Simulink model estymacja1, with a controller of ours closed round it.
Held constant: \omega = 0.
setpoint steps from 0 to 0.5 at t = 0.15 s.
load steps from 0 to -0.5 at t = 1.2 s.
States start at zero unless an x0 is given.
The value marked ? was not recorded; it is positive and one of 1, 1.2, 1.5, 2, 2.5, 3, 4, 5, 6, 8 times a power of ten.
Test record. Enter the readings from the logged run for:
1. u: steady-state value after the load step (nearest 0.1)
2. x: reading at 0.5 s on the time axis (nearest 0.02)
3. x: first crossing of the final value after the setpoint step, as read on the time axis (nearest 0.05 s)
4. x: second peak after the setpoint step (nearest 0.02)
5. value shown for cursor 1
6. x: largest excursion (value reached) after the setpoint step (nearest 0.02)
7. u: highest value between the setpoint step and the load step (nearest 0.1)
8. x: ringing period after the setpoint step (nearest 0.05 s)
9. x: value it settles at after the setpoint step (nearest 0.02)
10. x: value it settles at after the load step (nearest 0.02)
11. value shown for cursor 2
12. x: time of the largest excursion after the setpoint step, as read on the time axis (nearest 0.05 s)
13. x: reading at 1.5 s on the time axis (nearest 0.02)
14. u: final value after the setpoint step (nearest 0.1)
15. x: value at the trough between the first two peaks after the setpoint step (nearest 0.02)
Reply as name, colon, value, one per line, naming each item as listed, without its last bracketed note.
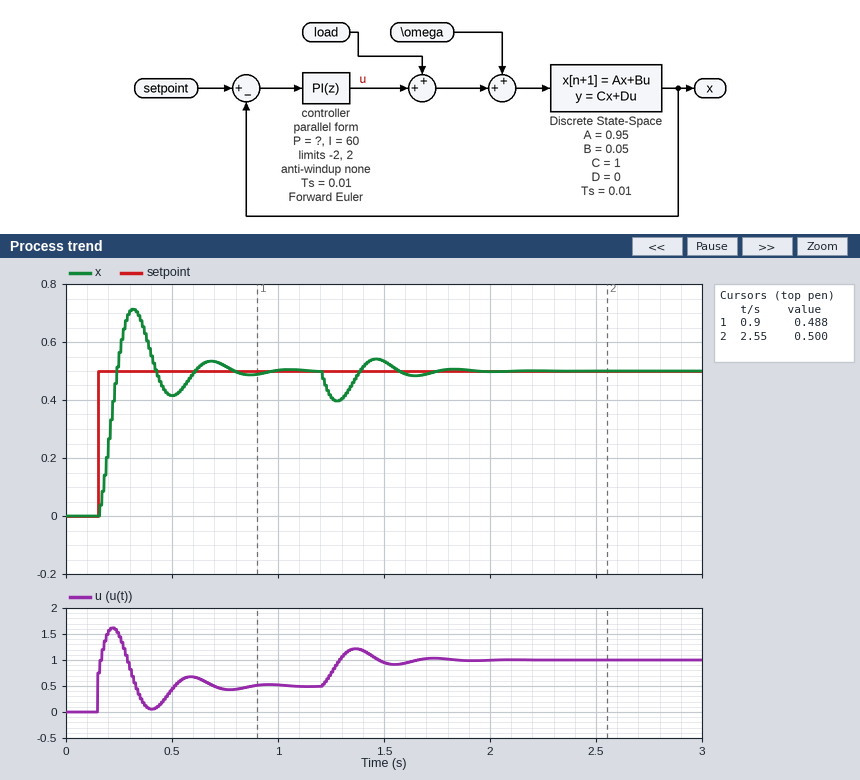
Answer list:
u: steady-state value after the load step: 1.0
x: reading at 0.5 s on the time axis: 0.42
x: first crossing of the final value after the setpoint step, as read on the time axis: 0.25 s
x: second peak after the setpoint step: 0.54
value shown for cursor 1: 0.488
x: largest excursion (value reached) after the setpoint step: 0.72
u: highest value between the setpoint step and the load step: 1.6
x: ringing period after the setpoint step: 0.35 s
x: value it settles at after the setpoint step: 0.50
x: value it settles at after the load step: 0.50
value shown for cursor 2: 0.500
x: time of the largest excursion after the setpoint step, as read on the time axis: 0.30 s
x: reading at 1.5 s on the time axis: 0.54
u: final value after the setpoint step: 0.5
x: value at the trough between the first two peaks after the setpoint step: 0.42
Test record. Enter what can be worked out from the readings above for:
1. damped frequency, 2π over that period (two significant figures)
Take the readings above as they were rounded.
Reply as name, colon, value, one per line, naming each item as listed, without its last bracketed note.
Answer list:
damped frequency, 2π over that period: 18 rad/s
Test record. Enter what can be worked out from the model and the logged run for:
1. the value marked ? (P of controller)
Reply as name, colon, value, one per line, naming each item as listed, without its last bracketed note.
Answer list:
the value marked ?: 1.5
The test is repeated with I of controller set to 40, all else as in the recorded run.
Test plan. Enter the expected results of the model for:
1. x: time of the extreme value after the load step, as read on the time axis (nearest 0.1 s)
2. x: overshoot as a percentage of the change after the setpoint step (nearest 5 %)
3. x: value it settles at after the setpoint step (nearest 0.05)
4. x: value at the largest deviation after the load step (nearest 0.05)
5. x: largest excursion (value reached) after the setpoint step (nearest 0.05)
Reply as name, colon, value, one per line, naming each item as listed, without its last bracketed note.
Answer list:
x: time of the extreme value after the load step, as read on the time axis: 1.3 s
x: overshoot as a percentage of the change after the setpoint step: 30 %
x: value it settles at after the setpoint step: 0.50
x: value at the largest deviation after the load step: 0.40
x: largest excursion (value reached) after the setpoint step: 0.65
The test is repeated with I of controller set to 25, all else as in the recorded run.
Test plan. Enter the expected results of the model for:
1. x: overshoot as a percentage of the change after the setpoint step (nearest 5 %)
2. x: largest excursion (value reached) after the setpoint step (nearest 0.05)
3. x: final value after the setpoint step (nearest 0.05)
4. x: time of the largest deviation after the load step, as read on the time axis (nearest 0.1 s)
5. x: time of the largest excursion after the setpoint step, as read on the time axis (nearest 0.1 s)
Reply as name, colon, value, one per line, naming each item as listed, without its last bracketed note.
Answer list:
x: overshoot as a percentage of the change after the setpoint step: 20 %
x: largest excursion (value reached) after the setpoint step: 0.60
x: final value after the setpoint step: 0.50
x: time of the largest deviation after the load step, as read on the time axis: 1.3 s
x: time of the largest excursion after the setpoint step, as read on the time axis: 0.4 s
